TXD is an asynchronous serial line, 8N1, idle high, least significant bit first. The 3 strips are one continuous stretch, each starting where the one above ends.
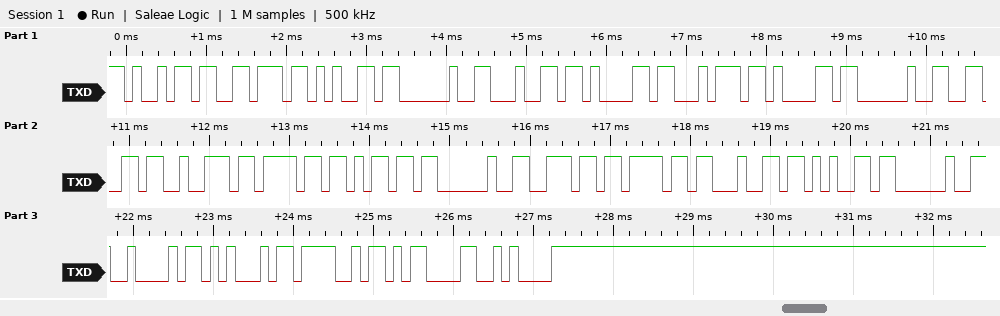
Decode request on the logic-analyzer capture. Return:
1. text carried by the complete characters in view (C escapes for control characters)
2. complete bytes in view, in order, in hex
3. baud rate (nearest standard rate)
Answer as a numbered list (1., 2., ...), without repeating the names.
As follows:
1. "ive data from node BEO\r\n"
2. 0x69 0x76 0x65 0x20 0x64 0x61 0x74 0x61 0x20 0x66 0x72 0x6F 0x6D 0x20 0x6E 0x6F 0x64 0x65 0x20 0x42 0x45 0x4F 0x0D 0x0A
3. 9600 baud
